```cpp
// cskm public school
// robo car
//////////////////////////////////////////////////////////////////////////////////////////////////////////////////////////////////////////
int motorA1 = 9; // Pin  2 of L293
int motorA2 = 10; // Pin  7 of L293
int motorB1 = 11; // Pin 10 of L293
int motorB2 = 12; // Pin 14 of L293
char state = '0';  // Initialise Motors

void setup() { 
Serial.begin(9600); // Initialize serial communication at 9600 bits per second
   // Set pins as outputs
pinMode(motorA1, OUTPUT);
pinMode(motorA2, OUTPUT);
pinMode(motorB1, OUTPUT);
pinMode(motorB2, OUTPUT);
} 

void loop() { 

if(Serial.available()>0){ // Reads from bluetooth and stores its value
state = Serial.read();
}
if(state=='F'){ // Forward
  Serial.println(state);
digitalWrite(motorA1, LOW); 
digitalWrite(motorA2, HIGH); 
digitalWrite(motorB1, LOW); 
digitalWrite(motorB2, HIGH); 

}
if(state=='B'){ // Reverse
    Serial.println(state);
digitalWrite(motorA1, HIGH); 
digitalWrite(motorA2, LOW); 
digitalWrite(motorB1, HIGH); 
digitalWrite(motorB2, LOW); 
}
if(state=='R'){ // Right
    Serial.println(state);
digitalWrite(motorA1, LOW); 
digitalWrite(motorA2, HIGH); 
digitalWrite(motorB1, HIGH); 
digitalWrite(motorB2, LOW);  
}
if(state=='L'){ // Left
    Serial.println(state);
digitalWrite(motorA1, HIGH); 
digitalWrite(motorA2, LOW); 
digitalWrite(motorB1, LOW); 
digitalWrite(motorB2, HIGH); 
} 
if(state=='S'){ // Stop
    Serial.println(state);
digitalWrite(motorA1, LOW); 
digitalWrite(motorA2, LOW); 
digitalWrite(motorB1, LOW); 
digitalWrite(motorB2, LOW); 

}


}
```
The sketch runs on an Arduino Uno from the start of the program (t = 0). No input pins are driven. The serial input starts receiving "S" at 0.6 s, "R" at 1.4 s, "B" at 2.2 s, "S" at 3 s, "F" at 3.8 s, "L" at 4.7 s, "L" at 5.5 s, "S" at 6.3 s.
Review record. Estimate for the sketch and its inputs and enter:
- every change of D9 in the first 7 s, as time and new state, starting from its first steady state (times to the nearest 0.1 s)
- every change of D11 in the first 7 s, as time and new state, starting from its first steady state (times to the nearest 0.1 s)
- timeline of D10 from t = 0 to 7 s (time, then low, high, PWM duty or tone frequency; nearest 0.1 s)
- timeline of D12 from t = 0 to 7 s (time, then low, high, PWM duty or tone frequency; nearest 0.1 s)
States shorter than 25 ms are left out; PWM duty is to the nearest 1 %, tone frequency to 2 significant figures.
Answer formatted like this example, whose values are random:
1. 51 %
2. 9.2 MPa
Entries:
1. 0 s low; 2.2 s high; 3 s low; 4.7 s high; 6.3 s low
2. 0 s low; 1.4 s high; 3 s low
3. 0 s low; 1.4 s high; 2.2 s low; 3.8 s high; 4.7 s low
4. 0 s low; 3.8 s high; 6.3 s low
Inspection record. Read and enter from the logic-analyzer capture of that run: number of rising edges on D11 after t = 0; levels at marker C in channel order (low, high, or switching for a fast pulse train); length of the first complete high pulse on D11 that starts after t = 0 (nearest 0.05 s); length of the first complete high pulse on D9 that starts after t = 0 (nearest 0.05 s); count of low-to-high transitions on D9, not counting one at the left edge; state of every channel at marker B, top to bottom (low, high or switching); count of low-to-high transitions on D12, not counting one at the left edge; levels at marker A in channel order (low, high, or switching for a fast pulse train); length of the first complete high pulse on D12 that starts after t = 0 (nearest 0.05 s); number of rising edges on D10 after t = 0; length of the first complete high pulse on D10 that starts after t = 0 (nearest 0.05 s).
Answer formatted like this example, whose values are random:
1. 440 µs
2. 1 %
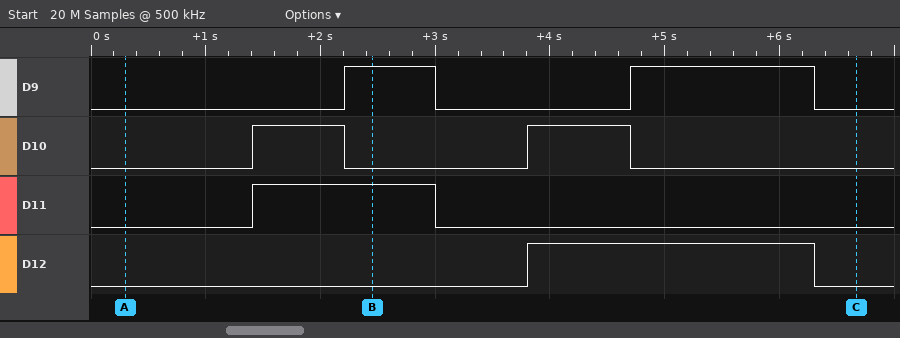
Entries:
1. 1
2. D9 low, D10 low, D11 low, D12 low
3. 1.60 s
4. 0.80 s
5. 2
6. D9 high, D10 low, D11 high, D12 low
7. 1
8. D9 low, D10 low, D11 low, D12 low
9. 2.50 s
10. 2
11. 0.80 s
